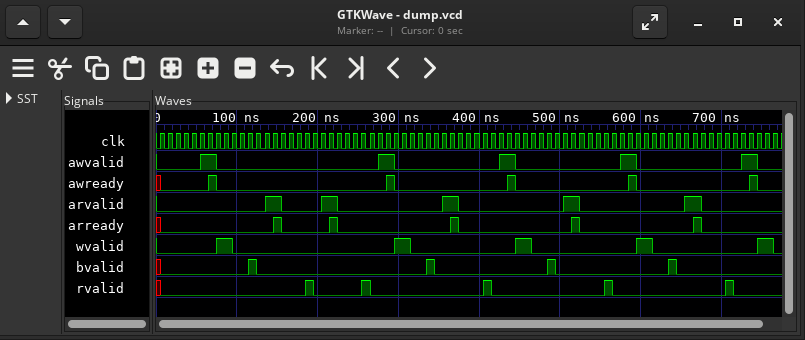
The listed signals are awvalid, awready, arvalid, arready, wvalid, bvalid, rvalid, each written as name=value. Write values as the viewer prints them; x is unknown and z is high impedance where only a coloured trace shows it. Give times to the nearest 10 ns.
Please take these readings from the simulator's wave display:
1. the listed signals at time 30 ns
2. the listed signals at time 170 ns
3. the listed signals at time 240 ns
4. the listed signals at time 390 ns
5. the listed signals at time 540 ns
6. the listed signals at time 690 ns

awvalid=0, awready=0, arvalid=0, arready=0, wvalid=0, bvalid=0, rvalid=0
awvalid=0, awready=0, arvalid=0, arready=0, wvalid=0, bvalid=0, rvalid=0
awvalid=0, awready=0, arvalid=0, arready=0, wvalid=0, bvalid=0, rvalid=0
awvalid=0, awready=0, arvalid=0, arready=0, wvalid=0, bvalid=0, rvalid=0
awvalid=0, awready=0, arvalid=0, arready=0, wvalid=0, bvalid=0, rvalid=0
awvalid=0, awready=0, arvalid=0, arready=0, wvalid=0, bvalid=0, rvalid=0
